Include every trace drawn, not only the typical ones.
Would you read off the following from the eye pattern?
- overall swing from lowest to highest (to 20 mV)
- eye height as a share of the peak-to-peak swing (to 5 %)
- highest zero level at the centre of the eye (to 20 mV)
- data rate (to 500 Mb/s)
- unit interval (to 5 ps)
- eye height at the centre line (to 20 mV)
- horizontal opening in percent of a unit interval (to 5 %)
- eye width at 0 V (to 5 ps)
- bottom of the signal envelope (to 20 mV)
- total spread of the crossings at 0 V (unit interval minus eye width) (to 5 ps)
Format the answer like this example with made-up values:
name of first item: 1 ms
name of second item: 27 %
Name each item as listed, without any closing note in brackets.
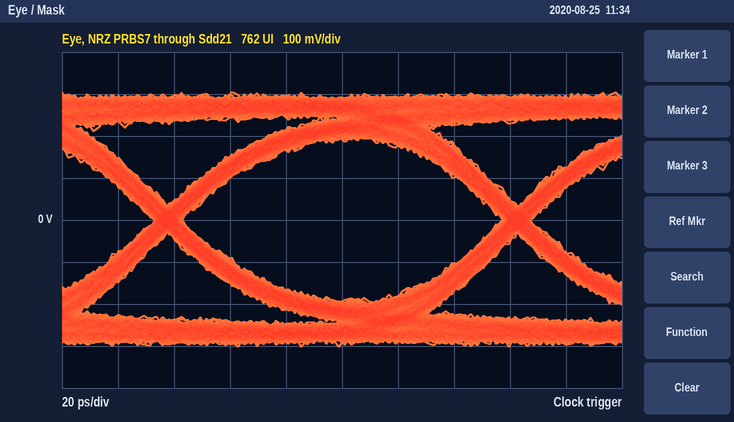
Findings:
overall swing from lowest to highest: 600 mV
eye height as a share of the peak-to-peak swing: 65 %
highest zero level at the centre of the eye: -200 mV
data rate: 8.0 Gb/s
unit interval: 125 ps
eye height at the centre line: 380 mV
horizontal opening in percent of a unit interval: 90 %
eye width at 0 V: 115 ps
bottom of the signal envelope: -300 mV
total spread of the crossings at 0 V (unit interval minus eye width): 10 ps
